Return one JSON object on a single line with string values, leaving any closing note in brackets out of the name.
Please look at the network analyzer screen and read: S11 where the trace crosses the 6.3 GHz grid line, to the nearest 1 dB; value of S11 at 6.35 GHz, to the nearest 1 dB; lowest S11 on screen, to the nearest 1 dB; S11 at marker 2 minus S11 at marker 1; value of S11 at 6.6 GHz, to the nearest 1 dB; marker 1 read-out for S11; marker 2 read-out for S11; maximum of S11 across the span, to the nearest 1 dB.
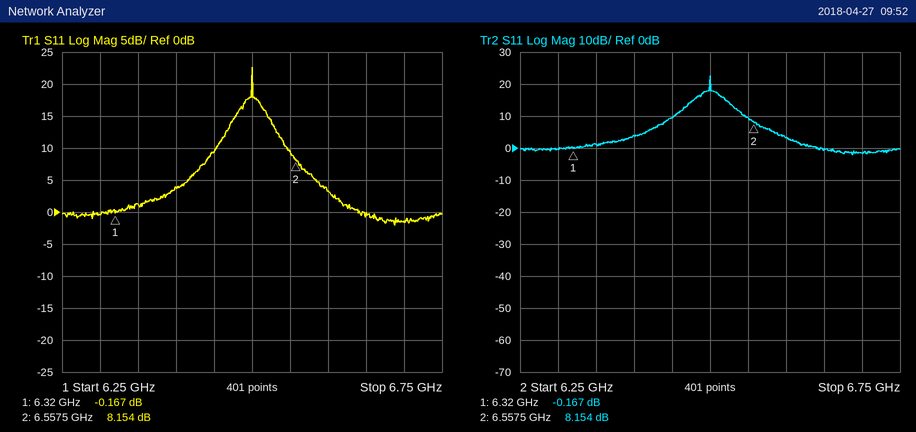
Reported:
{"S11 where the trace crosses the 6.3 GHz grid line, to the nearest 1 dB": "0 dB", "value of S11 at 6.35 GHz, to the nearest 1 dB": "1 dB", "lowest S11 on screen, to the nearest 1 dB": "-2 dB", "S11 at marker 2 minus S11 at marker 1": "8.321 dB", "value of S11 at 6.6 GHz, to the nearest 1 dB": "3 dB", "marker 1 read-out for S11": "-0.167 dB", "marker 2 read-out for S11": "8.154 dB", "maximum of S11 across the span, to the nearest 1 dB": "23 dB"}
